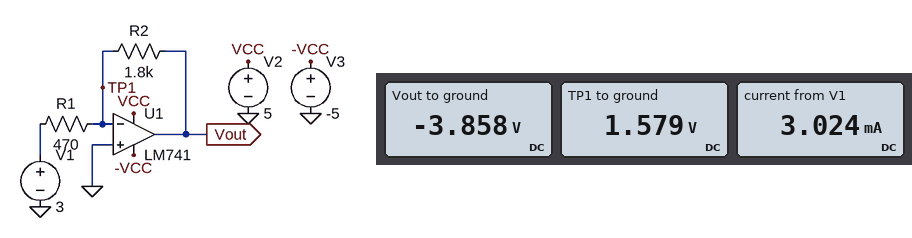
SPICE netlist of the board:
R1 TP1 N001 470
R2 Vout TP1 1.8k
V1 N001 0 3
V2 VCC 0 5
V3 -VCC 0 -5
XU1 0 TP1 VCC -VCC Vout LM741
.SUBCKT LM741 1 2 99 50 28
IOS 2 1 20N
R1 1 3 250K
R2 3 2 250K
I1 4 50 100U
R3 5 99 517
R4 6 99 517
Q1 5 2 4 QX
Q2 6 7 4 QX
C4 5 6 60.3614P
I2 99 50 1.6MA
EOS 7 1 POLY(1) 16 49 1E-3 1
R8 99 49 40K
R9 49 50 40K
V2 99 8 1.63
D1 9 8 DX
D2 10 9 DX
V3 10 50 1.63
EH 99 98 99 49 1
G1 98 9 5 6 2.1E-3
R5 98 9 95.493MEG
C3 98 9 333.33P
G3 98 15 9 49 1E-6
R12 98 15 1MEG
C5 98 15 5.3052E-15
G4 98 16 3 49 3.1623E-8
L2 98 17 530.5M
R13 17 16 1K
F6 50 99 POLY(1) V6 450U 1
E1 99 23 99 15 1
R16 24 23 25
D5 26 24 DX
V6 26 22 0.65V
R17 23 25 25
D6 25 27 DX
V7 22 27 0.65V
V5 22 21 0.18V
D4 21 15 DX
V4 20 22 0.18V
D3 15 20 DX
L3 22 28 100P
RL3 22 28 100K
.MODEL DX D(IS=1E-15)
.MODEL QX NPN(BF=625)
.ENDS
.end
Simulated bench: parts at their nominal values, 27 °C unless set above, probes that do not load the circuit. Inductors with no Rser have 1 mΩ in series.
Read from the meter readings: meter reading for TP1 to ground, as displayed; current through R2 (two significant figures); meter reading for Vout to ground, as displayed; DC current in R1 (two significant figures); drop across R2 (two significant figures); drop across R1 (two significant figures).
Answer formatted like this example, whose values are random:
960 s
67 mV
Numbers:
1.579 V
3.0 mA
-3.858 V
3.0 mA
5.4 V
1.4 V
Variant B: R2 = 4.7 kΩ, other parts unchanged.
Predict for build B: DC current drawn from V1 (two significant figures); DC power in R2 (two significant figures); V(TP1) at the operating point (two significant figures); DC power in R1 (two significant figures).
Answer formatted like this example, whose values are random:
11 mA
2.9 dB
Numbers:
1.3 mA
8.4 mW
2.4 V
850 µW
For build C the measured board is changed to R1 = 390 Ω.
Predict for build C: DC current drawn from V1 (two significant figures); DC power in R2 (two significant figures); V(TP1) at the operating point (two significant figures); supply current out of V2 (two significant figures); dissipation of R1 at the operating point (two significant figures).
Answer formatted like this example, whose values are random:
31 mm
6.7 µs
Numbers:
3.1 mA
18 mW
1.8 V
1.3 mA
3.8 mW
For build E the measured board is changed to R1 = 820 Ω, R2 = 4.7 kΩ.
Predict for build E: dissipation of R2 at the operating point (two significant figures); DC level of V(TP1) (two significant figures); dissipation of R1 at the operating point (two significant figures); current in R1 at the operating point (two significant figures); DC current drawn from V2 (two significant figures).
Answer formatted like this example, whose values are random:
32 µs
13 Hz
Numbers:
7.4 mW
2.0 V
1.3 mW
1.3 mA
1.3 mA
